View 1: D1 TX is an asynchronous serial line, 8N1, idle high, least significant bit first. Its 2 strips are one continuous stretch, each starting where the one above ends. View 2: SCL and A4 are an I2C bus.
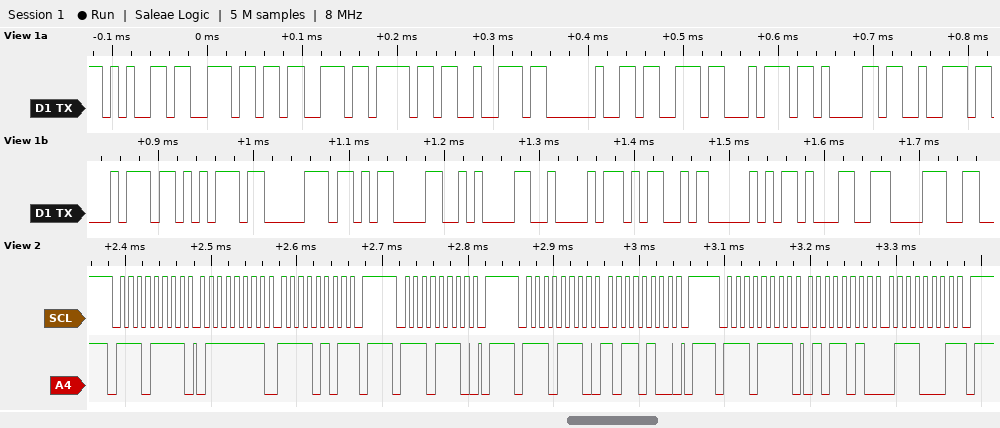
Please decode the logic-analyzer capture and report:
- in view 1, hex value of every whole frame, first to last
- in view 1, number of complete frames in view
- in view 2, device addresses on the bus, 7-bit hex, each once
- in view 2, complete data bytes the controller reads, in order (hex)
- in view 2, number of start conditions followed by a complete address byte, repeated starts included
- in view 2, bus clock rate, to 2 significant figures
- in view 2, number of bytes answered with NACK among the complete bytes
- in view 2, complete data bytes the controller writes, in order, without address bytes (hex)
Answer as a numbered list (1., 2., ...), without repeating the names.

1. 65 6E 73 6F 72 20 73 74 61 72 74 75 70 0D 0A 42 4D 50 31 38
2. 20
3. 0x77
4. 7F F5 5A 71
5. 4
6. 100 kHz
7. 2
8. B4
